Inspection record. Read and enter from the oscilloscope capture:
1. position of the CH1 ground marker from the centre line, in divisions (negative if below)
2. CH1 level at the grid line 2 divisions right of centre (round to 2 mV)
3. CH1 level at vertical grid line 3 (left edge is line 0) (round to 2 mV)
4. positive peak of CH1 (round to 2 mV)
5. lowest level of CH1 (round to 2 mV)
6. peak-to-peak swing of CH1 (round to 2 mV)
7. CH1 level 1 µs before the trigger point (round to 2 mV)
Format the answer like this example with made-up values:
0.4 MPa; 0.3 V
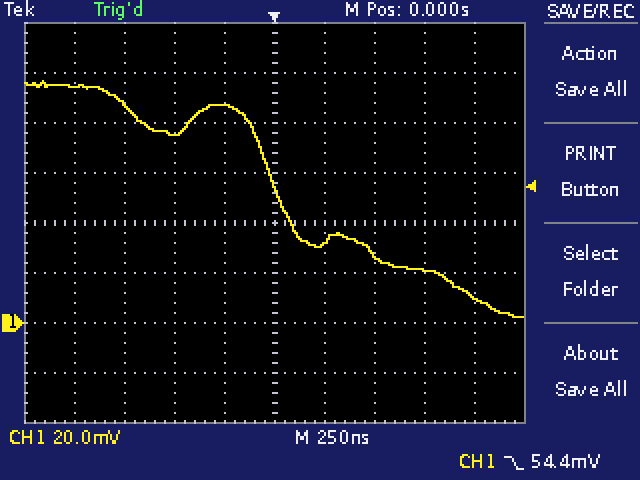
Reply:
-2.0 div; 28 mV; 76 mV; 96 mV; 2 mV; 94 mV; 94 mV
